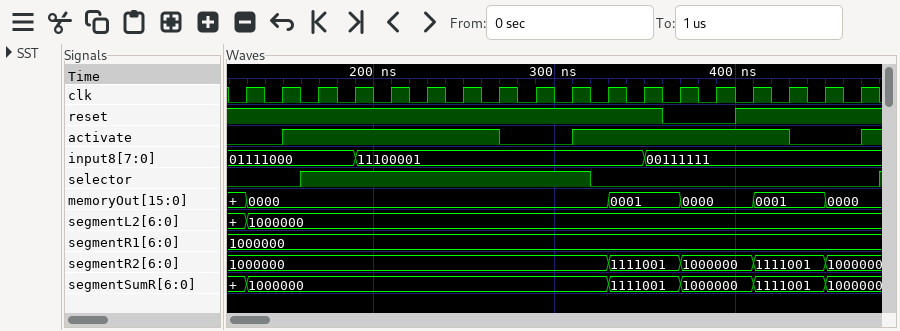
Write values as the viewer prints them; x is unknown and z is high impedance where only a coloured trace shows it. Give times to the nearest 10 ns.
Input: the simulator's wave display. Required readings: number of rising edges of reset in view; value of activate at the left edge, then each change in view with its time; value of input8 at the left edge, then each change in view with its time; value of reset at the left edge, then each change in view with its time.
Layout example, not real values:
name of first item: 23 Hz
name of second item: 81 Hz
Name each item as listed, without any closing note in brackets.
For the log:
number of rising edges of reset in view: 1
value of activate at the left edge, then each change in view with its time: 0, 1 at 150 ns, 0 at 270 ns, 1 at 310 ns, 0 at 430 ns, 1 at 470 ns
value of input8 at the left edge, then each change in view with its time: 01111000, 11100001 at 190 ns, 00111111 at 350 ns
value of reset at the left edge, then each change in view with its time: 1, 0 at 360 ns, 1 at 400 ns
